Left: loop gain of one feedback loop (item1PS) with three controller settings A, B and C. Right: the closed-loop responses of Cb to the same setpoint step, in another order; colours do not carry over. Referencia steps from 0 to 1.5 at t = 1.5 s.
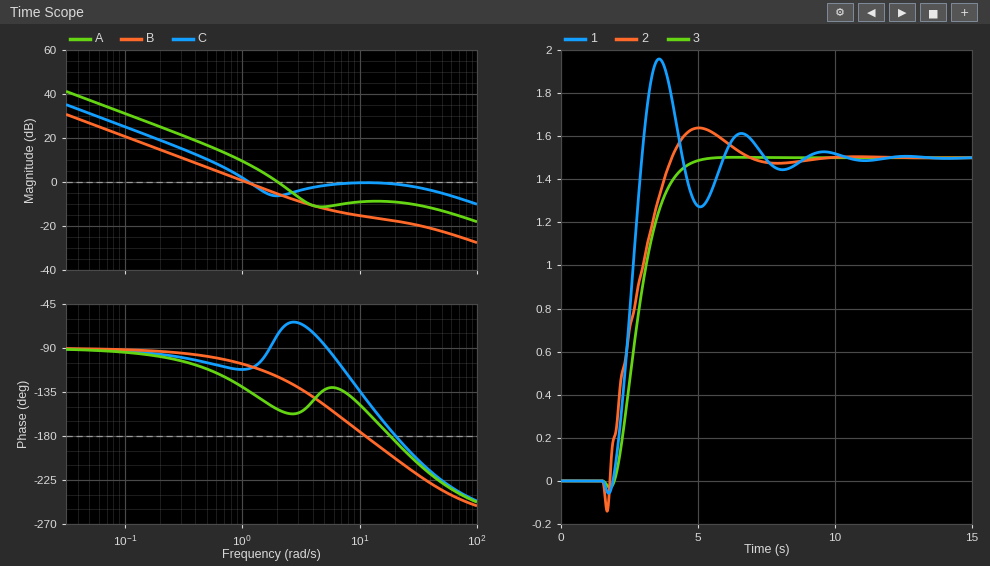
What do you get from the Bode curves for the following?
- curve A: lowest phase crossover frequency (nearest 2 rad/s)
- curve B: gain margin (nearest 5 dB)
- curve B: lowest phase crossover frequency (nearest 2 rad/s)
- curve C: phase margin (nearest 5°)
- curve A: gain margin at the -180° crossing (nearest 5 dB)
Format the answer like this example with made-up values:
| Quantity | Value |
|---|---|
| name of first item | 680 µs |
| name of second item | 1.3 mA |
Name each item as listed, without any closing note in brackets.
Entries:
| Quantity | Value |
|---|---|
| curve A: lowest phase crossover frequency | 18 rad/s |
| curve B: gain margin | 15 dB |
| curve B: lowest phase crossover frequency | 12 rad/s |
| curve C: phase margin | 70° |
| curve A: gain margin at the -180° crossing | 10 dB |
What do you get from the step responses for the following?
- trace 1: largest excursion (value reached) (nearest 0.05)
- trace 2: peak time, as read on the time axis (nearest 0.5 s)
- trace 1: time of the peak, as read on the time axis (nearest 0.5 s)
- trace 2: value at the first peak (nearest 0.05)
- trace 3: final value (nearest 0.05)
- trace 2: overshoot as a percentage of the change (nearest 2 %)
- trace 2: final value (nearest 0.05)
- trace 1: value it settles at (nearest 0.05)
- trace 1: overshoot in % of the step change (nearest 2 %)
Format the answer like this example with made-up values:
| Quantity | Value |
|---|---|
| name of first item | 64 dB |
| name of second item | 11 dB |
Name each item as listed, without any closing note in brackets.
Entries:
| Quantity | Value |
|---|---|
| trace 1: largest excursion (value reached) | 1.95 |
| trace 2: peak time, as read on the time axis | 5.0 s |
| trace 1: time of the peak, as read on the time axis | 3.5 s |
| trace 2: value at the first peak | 1.65 |
| trace 3: final value | 1.50 |
| trace 2: overshoot as a percentage of the change | 10 % |
| trace 2: final value | 1.50 |
| trace 1: value it settles at | 1.50 |
| trace 1: overshoot in % of the step change | 30 % |
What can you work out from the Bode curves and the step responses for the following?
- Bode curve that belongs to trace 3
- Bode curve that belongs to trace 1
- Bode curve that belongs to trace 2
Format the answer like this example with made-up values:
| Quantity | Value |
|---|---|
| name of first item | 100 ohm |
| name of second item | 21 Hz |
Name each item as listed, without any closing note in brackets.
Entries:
| Quantity | Value |
|---|---|
| Bode curve that belongs to trace 3 | B |
| Bode curve that belongs to trace 1 | A |
| Bode curve that belongs to trace 2 | C |
